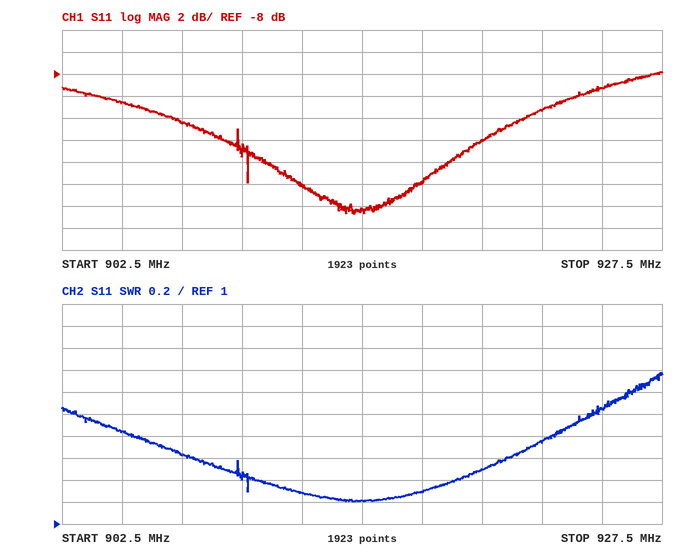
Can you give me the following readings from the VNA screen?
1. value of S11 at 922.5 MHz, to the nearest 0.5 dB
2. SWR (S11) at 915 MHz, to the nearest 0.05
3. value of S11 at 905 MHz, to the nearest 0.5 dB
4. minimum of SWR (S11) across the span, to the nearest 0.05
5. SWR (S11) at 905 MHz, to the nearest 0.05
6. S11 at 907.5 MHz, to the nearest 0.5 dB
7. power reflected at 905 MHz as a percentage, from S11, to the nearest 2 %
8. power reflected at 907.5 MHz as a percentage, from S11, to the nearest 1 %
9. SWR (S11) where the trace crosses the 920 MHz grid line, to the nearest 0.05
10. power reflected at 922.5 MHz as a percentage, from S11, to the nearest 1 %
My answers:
-11.5 dB
1.20
-10.5 dB
1.20
1.85
-12.5 dB
8 %
6 %
1.50
7 %
